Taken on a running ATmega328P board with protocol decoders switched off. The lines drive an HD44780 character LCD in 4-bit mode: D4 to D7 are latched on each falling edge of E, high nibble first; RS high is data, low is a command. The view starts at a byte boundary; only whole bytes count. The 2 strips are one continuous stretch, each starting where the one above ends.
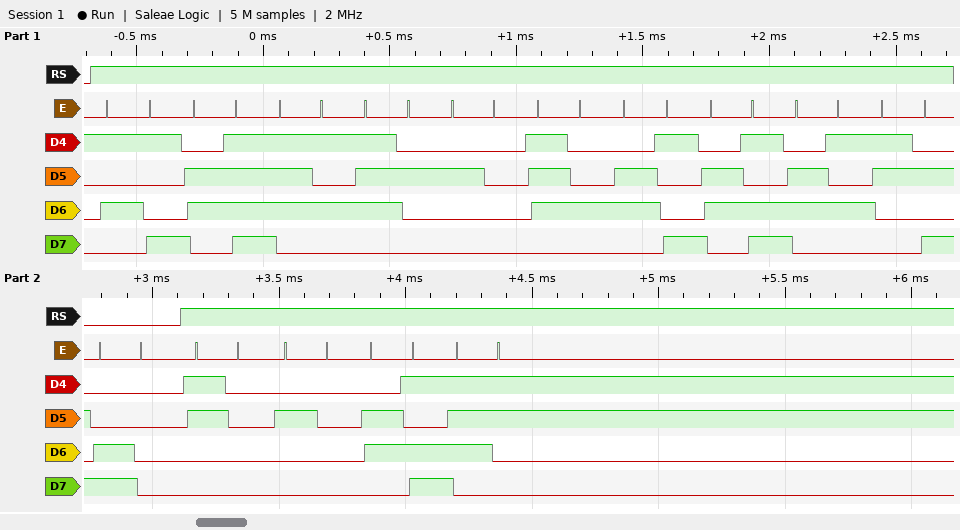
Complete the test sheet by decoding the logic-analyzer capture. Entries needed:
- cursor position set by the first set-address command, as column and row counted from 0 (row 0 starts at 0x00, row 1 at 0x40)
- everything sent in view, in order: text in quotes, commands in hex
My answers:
column 0, row 1
"Your time:" 0xC0 "0 ms"
